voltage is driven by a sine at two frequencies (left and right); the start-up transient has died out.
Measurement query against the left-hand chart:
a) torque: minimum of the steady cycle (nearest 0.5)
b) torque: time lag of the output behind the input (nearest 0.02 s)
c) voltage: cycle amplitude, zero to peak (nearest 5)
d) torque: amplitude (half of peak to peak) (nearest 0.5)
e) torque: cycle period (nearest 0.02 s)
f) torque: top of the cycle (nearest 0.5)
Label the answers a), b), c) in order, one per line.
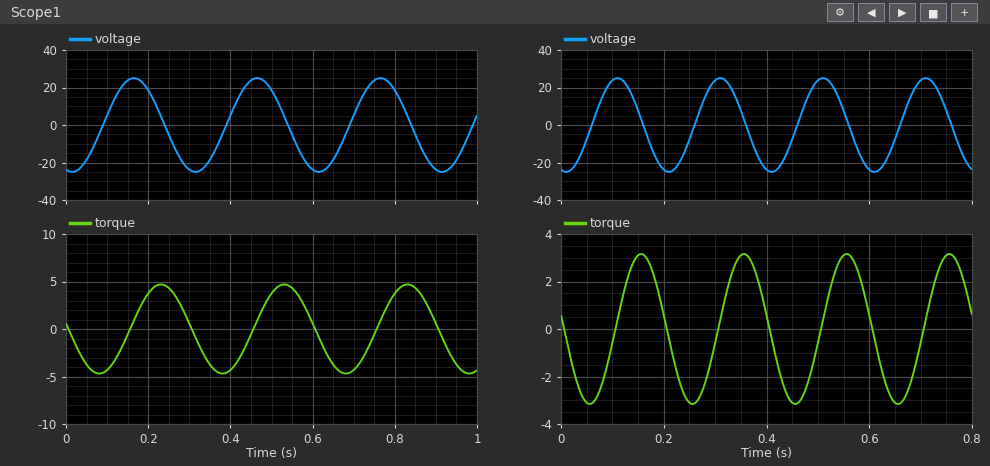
a) -4.5
b) 0.06 s
c) 25
d) 4.5
e) 0.30 s
f) 4.5
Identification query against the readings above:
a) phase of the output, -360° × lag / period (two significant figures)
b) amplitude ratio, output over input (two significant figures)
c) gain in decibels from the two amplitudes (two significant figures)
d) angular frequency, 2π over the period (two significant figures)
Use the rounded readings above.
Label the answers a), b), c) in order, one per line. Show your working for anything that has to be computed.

a) -360 × 0.06 / 0.3 = -72°
b) 4.5 / 25 = 0.18
c) 20 log10(4.5 / 25) = -15 dB
d) 2π / 0.3 = 21 rad/s
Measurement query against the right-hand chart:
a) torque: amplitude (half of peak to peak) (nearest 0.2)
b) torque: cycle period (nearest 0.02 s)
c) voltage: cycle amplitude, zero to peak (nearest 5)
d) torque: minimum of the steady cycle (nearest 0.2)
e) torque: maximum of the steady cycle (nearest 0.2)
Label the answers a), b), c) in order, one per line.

a) 3.2
b) 0.20 s
c) 25
d) -3.2
e) 3.2
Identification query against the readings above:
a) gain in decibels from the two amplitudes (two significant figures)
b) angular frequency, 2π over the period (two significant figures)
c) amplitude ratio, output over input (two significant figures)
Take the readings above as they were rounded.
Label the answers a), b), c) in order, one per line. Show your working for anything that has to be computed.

a) 20 log10(3.2 / 25) = -18 dB
b) 2π / 0.2 = 31 rad/s
c) 3.2 / 25 = 0.13
